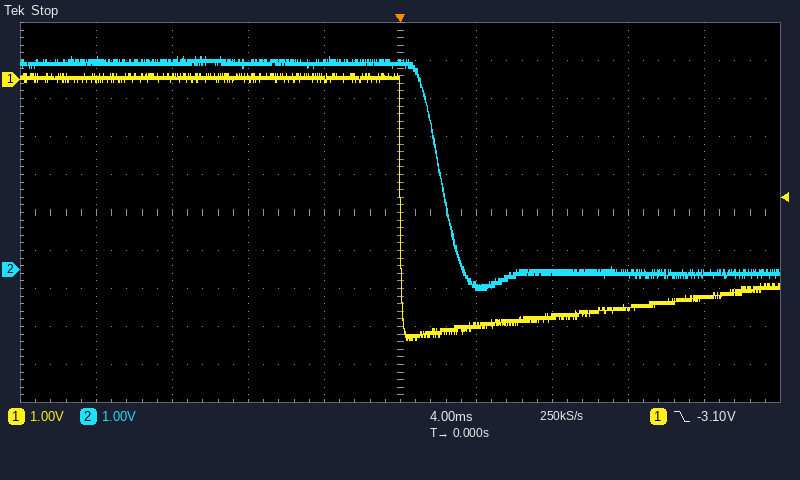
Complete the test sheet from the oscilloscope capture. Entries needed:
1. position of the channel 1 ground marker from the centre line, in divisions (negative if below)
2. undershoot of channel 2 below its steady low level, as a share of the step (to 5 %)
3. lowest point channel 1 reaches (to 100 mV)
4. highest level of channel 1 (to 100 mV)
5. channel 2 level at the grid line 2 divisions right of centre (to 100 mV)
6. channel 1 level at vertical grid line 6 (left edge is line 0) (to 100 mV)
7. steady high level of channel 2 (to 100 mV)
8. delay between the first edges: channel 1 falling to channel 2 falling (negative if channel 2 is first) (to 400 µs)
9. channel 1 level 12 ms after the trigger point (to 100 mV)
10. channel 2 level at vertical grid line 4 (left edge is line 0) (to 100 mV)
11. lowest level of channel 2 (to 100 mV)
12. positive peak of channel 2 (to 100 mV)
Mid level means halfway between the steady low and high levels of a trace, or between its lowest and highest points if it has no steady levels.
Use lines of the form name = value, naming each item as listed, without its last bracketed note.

position of the channel 1 ground marker from the centre line, in divisions = +3.5 div
undershoot of channel 2 below its steady low level, as a share of the step = 10 %
lowest point channel 1 reaches = -6.9 V
highest level of channel 1 = 200 mV
channel 2 level at the grid line 2 divisions right of centre = -100 mV
channel 1 level at vertical grid line 6 (left edge is line 0) = -6.5 V
steady high level of channel 2 = 5.4 V
delay between the first edges: channel 1 falling to channel 2 falling (negative if channel 2 is first) = +2.0 ms
channel 1 level 12 ms after the trigger point = -6.0 V
channel 2 level at vertical grid line 4 (left edge is line 0) = 5.4 V
lowest level of channel 2 = -600 mV
positive peak of channel 2 = 5.6 V
